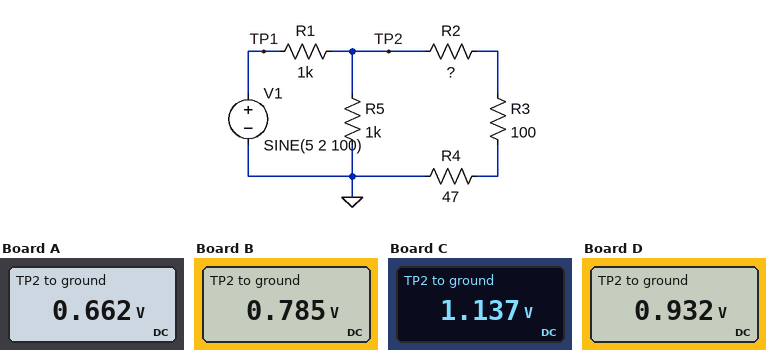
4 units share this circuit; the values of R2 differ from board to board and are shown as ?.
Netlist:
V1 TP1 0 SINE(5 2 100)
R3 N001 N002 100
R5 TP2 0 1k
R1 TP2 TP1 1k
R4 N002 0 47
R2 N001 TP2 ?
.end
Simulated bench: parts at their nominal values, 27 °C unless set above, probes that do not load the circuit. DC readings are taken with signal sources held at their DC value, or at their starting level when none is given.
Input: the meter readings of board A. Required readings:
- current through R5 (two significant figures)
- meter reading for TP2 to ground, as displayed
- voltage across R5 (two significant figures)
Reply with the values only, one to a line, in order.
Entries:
660 µA
0.662 V
660 mV
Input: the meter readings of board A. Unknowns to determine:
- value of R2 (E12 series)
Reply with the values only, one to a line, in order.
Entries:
33 Ω
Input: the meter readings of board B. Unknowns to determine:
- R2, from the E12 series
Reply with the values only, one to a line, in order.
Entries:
82 Ω
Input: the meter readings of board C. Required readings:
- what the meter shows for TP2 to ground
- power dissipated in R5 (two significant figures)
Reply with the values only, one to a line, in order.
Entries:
1.137 V
1.3 mW
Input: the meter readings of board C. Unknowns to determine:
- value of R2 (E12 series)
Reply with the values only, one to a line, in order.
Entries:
270 Ω
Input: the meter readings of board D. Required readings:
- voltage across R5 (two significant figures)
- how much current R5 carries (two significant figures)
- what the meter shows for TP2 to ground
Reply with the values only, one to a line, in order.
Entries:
930 mV
930 µA
0.932 V
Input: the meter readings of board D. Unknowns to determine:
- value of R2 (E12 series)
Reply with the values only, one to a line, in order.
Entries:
150 Ω
